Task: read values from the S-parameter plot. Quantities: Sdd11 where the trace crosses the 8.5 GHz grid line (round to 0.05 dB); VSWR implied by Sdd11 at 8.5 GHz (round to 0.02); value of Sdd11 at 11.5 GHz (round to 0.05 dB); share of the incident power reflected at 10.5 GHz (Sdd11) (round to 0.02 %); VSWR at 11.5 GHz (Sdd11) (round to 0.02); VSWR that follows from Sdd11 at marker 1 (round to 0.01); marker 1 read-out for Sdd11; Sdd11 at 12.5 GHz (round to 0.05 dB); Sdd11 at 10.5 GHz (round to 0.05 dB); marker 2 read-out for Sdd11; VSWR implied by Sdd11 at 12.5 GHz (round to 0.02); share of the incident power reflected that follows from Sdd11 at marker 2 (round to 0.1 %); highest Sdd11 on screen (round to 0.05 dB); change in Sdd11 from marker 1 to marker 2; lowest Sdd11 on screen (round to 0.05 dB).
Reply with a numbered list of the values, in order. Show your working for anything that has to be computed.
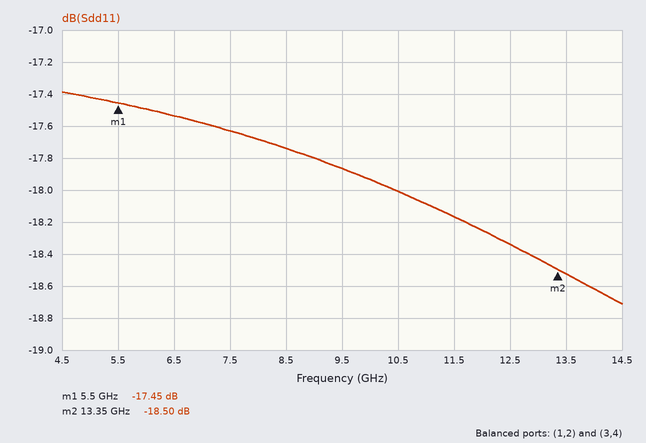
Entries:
1. -17.75 dB
2. |Γ| = 10^(-17.75/20) = 0.1296; VSWR = (1 + 0.1296)/(1 − 0.1296) ≈ 1.30
3. -18.15 dB
4. 10^(-18/10) ≈ 1.58 %
5. |Γ| = 10^(-18.15/20) = 0.1237; VSWR = (1 + 0.1237)/(1 − 0.1237) ≈ 1.28
6. (1 + 0.1341)/(1 − 0.1341) ≈ 1.31
7. -17.45 dB
8. -18.35 dB
9. -18.00 dB
10. -18.50 dB
11. |Γ| = 10^(-18.35/20) = 0.1209; VSWR = (1 + 0.1209)/(1 − 0.1209) ≈ 1.28
12. 10^(-18.5/10) ≈ 1.4 %
13. -17.40 dB
14. -18.5 − (-17.45) = -1.05 dB
15. -18.70 dB
